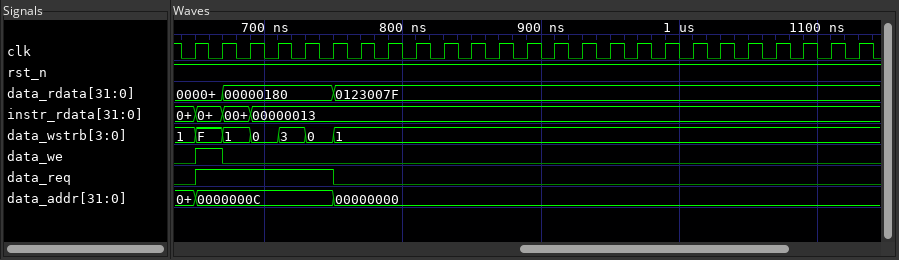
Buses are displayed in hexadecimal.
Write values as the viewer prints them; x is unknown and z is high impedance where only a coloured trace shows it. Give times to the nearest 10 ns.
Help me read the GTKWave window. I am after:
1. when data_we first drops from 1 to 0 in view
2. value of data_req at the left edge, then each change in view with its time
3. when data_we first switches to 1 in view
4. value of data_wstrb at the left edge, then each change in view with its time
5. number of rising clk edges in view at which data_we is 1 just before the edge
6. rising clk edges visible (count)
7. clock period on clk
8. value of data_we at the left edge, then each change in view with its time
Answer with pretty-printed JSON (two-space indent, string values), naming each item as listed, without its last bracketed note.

{
  "when data_we first drops from 1 to 0 in view": "670 ns",
  "value of data_req at the left edge, then each change in view with its time": "0, 1 at 650 ns, 0 at 750 ns",
  "when data_we first switches to 1 in view": "650 ns",
  "value of data_wstrb at the left edge, then each change in view with its time": "1, F at 650 ns, 1 at 670 ns, 0 at 690 ns, 3 at 710 ns, 0 at 730 ns, 1 at 750 ns",
  "number of rising clk edges in view at which data_we is 1 just before the edge": "1",
  "rising clk edges visible": "25",
  "clock period on clk": "20 ns",
  "value of data_we at the left edge, then each change in view with its time": "0, 1 at 650 ns, 0 at 670 ns"
}
